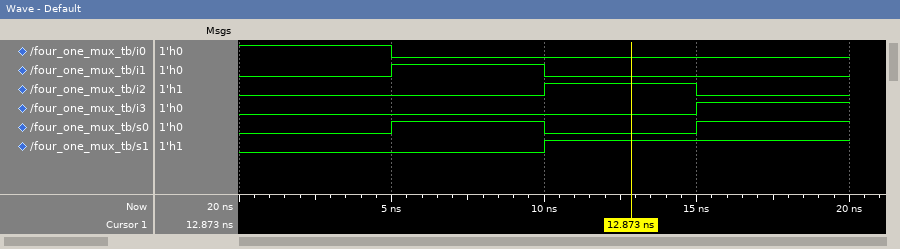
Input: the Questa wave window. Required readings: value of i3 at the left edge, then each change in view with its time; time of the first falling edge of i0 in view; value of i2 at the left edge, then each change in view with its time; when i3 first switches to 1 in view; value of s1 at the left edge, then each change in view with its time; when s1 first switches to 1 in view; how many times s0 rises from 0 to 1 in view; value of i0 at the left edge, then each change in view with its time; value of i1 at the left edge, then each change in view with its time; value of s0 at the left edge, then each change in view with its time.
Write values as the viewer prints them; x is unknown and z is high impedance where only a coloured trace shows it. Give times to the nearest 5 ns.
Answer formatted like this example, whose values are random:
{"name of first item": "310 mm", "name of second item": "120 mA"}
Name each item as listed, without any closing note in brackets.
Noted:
{"value of i3 at the left edge, then each change in view with its time": "0, 1 at 15 ns", "time of the first falling edge of i0 in view": "5 ns", "value of i2 at the left edge, then each change in view with its time": "0, 1 at 10 ns, 0 at 15 ns", "when i3 first switches to 1 in view": "15 ns", "value of s1 at the left edge, then each change in view with its time": "0, 1 at 10 ns", "when s1 first switches to 1 in view": "10 ns", "how many times s0 rises from 0 to 1 in view": "2", "value of i0 at the left edge, then each change in view with its time": "1, 0 at 5 ns", "value of i1 at the left edge, then each change in view with its time": "0, 1 at 5 ns, 0 at 10 ns", "value of s0 at the left edge, then each change in view with its time": "0, 1 at 5 ns, 0 at 10 ns, 1 at 15 ns"}
